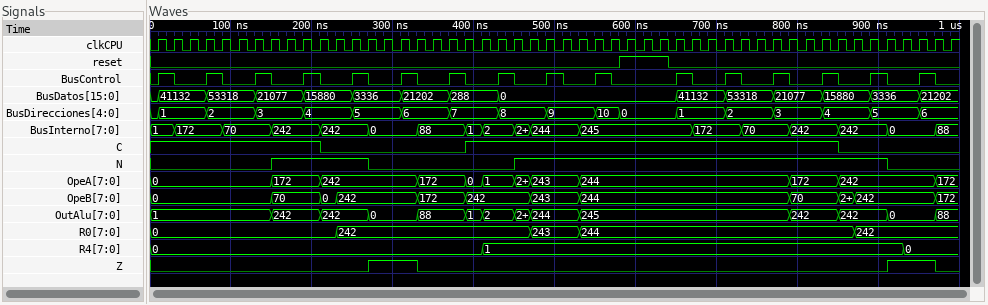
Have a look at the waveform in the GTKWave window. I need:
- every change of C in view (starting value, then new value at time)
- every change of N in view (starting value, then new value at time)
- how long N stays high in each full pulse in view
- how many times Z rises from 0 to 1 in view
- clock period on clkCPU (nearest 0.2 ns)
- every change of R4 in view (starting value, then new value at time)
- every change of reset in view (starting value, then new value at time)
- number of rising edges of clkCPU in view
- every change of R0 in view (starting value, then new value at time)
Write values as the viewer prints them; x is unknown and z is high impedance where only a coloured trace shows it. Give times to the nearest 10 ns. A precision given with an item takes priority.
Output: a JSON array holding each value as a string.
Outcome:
["1, 0 at 210 ns, 1 at 390 ns, 0 at 850 ns", "0, 1 at 150 ns, 0 at 270 ns, 1 at 450 ns, 0 at 910 ns", "120 ns, 460 ns", "2", "20 ns", "0, 1 at 410 ns, 0 at 930 ns", "0, 1 at 580 ns, 0 at 640 ns", "50", "0, 242 at 230 ns, 243 at 470 ns, 244 at 530 ns, 242 at 870 ns"]
